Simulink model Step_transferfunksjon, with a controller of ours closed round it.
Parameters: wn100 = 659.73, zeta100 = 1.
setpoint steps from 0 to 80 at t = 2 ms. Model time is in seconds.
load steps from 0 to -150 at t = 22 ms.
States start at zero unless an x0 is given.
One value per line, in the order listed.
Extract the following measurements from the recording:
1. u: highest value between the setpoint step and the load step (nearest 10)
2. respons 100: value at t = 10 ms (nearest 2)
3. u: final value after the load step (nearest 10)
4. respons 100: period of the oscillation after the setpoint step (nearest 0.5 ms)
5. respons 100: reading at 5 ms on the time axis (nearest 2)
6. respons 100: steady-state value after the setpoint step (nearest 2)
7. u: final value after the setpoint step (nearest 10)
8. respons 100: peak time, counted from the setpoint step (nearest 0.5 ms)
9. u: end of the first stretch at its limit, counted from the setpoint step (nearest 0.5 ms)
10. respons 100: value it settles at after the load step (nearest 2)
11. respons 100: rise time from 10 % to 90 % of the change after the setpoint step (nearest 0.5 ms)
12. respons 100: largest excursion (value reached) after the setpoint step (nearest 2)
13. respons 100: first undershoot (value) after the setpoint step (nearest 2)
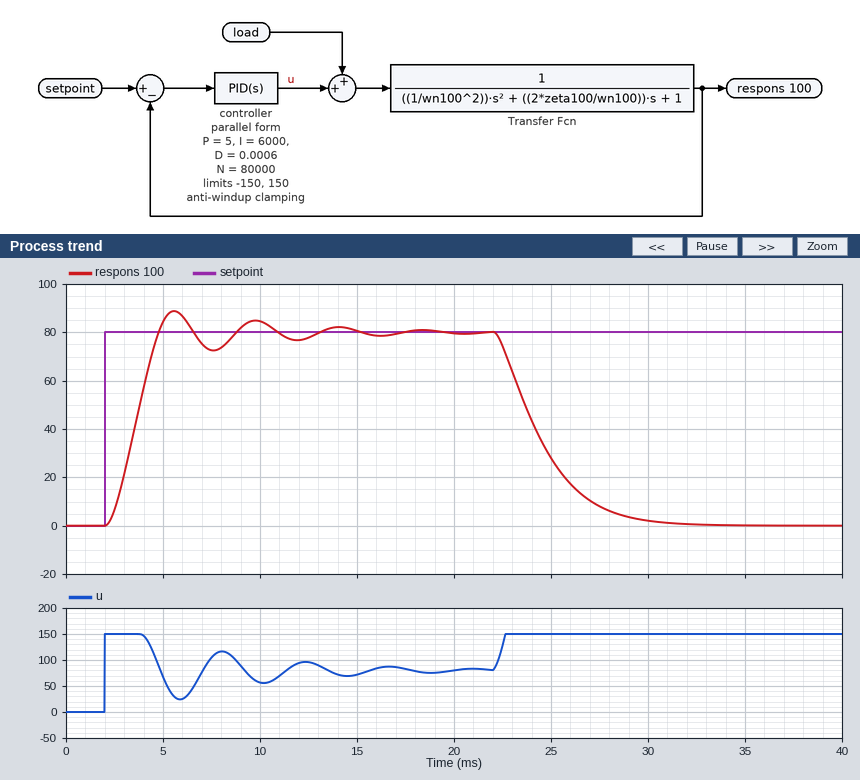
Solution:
150
84
150
4.0 ms
84
80
80
3.5 ms
2.0 ms
0
2.0 ms
88
72
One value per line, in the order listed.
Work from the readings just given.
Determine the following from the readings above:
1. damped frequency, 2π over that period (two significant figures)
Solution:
1.6 rad/ms
